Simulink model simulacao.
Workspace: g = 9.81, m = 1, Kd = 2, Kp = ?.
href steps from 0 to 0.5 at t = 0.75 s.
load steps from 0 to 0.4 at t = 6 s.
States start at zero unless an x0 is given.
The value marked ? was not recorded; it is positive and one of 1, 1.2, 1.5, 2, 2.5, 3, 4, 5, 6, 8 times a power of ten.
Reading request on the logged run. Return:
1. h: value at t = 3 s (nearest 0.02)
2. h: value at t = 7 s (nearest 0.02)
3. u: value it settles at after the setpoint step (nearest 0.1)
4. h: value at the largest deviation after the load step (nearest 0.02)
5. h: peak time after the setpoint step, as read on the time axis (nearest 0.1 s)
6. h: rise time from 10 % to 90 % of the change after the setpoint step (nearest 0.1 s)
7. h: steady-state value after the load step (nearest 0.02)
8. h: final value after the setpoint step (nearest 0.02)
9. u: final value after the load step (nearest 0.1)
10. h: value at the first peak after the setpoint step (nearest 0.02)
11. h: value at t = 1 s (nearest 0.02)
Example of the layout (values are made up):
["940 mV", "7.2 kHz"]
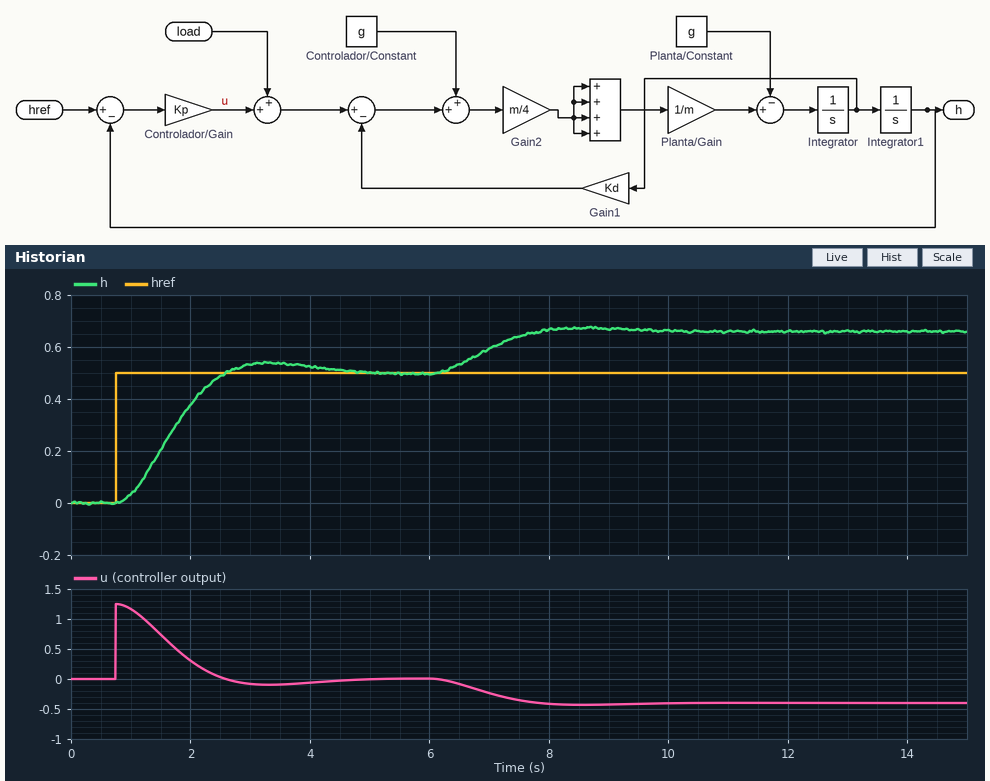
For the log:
["0.54", "0.60", "0.0", "0.68", "3.3 s", "1.2 s", "0.66", "0.50", "-0.4", "0.54", "0.04"]
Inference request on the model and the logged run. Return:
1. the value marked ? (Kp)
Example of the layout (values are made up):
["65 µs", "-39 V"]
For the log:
["2.5"]
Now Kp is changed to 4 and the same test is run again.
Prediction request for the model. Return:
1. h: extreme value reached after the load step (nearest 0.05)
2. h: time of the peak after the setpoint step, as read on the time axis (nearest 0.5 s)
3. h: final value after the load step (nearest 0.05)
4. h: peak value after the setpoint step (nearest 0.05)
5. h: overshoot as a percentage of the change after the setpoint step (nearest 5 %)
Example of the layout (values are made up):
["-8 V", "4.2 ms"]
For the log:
["0.60", "2.5 s", "0.60", "0.60", "15 %"]
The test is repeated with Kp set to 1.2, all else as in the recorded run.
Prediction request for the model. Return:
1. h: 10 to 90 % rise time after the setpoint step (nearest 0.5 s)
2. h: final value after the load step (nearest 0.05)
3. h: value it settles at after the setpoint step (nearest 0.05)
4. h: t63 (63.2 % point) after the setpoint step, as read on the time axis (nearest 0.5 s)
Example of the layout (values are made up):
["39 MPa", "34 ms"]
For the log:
["2.5 s", "0.85", "0.50", "2.5 s"]
